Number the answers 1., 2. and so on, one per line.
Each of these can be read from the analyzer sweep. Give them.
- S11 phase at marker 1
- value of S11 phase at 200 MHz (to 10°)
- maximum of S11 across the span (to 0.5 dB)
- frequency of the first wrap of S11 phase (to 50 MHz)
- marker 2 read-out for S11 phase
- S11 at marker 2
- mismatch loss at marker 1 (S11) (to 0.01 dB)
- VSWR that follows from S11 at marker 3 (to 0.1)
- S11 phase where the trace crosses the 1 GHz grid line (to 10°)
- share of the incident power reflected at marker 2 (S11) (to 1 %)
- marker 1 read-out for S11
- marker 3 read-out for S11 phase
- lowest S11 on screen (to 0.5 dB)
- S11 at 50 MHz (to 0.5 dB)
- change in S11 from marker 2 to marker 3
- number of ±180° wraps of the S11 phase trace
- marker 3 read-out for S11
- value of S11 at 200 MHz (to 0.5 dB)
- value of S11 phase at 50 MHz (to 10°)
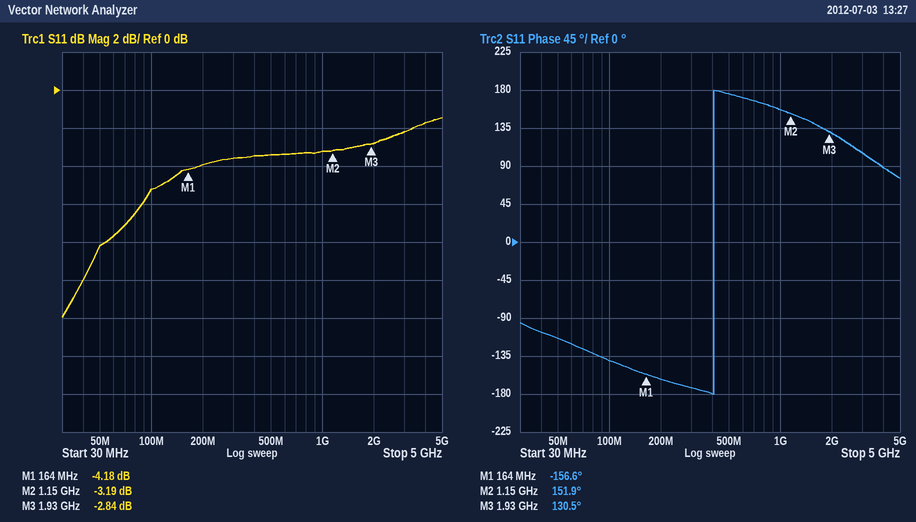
1. -156.6°
2. -160°
3. -1.5 dB
4. 400 MHz
5. 151.9°
6. -3.19 dB
7. 2.09 dB
8. 6.2
9. 160°
10. 48 %
11. -4.18 dB
12. 130.5°
13. -12.0 dB
14. -8.0 dB
15. 0.35 dB
16. 1
17. -2.84 dB
18. -4.0 dB
19. -110°
